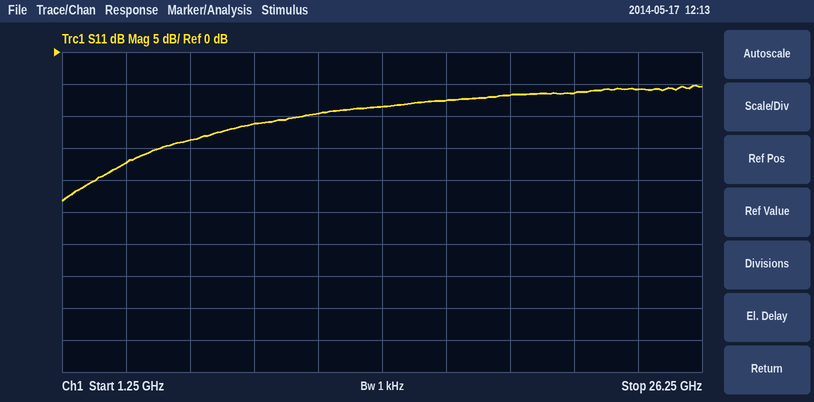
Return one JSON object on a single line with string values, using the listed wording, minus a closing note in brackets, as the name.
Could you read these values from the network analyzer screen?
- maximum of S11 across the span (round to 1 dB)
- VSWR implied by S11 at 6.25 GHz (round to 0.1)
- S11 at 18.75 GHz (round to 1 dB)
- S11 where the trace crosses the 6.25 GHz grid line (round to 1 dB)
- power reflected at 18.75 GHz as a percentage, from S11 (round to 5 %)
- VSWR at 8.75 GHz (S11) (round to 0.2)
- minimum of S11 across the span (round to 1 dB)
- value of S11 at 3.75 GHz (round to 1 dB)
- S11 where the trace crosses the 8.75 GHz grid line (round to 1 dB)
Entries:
{"maximum of S11 across the span": "-5 dB", "VSWR implied by S11 at 6.25 GHz": "1.5", "S11 at 18.75 GHz": "-7 dB", "S11 where the trace crosses the 6.25 GHz grid line": "-14 dB", "power reflected at 18.75 GHz as a percentage, from S11": "20 %", "VSWR at 8.75 GHz (S11)": "1.8", "minimum of S11 across the span": "-23 dB", "value of S11 at 3.75 GHz": "-17 dB", "S11 where the trace crosses the 8.75 GHz grid line": "-11 dB"}
